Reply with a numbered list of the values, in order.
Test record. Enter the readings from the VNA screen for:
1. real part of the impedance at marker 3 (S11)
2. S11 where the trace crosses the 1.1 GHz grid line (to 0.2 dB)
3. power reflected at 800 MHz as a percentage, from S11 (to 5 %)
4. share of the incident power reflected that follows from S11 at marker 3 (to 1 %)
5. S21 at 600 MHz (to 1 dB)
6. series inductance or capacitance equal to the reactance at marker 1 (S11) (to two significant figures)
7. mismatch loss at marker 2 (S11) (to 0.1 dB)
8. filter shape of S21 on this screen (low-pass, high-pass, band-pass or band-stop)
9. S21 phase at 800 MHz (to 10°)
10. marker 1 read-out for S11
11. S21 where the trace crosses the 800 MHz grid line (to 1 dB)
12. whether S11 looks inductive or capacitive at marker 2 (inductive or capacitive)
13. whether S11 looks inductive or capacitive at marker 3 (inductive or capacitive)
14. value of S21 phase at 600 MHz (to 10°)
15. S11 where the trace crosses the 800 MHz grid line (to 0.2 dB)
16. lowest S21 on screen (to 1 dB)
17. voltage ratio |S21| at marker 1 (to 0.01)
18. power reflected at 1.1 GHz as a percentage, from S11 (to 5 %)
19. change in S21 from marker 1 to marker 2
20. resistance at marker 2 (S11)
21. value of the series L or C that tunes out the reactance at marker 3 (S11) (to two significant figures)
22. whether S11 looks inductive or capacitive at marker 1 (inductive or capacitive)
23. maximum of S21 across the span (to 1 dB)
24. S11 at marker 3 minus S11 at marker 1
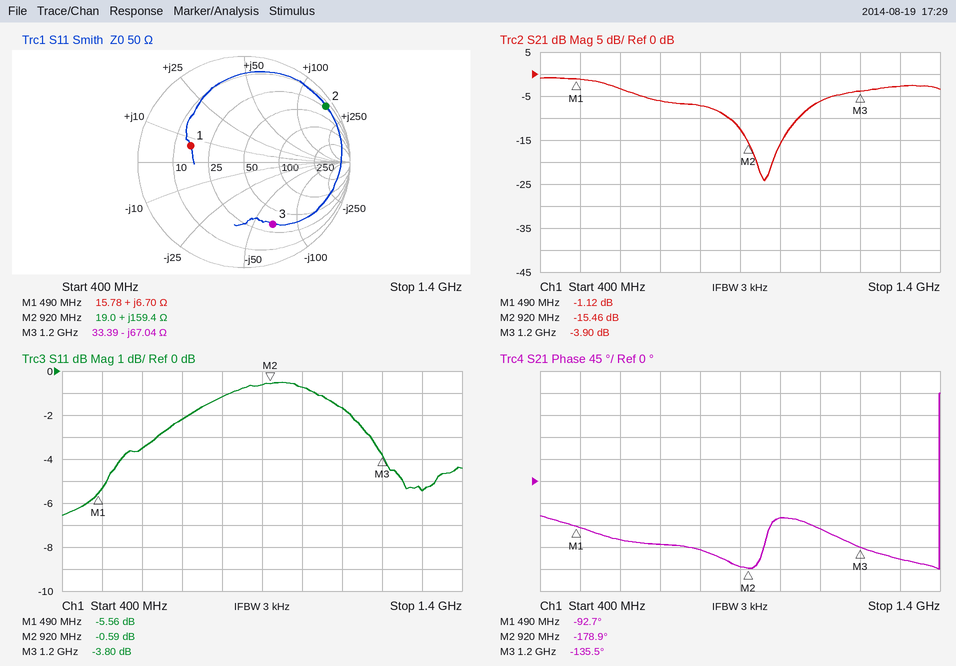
1. 33.39 Ω
2. -1.6 dB
3. 75 %
4. 42 %
5. -3 dB
6. 2.2 nH
7. 9.0 dB
8. band-stop
9. -140°
10. -5.56 dB
11. -7 dB
12. inductive
13. capacitive
14. -120°
15. -1.2 dB
16. -24 dB
17. 0.88
18. 70 %
19. -14.34 dB
20. 19.0 Ω
21. 8.9 nH
22. inductive
23. -1 dB
24. 1.76 dB
